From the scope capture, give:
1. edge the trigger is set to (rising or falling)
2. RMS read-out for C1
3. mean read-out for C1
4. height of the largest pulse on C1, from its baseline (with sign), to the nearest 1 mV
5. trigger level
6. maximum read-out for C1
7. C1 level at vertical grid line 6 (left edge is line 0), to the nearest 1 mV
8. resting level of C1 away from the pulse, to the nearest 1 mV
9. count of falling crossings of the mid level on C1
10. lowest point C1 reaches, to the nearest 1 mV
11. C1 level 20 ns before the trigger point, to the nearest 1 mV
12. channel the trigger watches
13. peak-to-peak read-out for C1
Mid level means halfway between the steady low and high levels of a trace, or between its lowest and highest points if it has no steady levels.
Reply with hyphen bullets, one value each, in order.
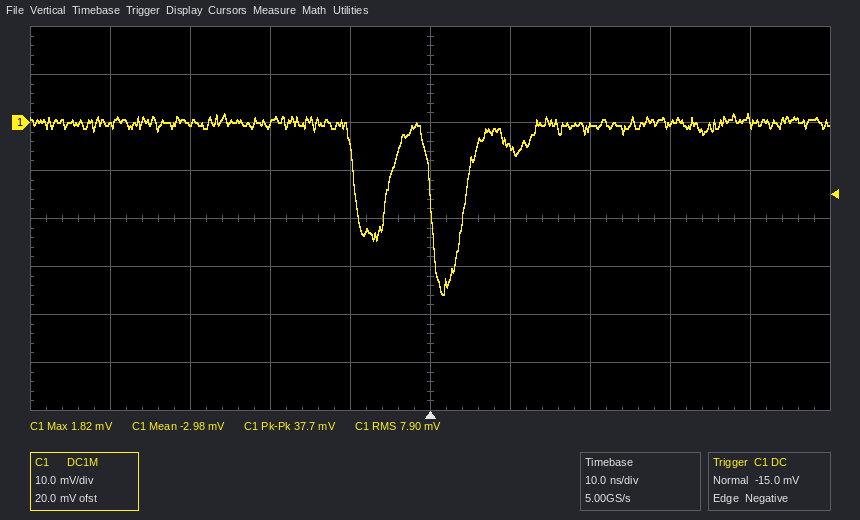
- falling
- 7.90 mV
- -2.98 mV
- -36 mV
- -15.0 mV
- 1.82 mV
- -5 mV
- 0 mV
- 2
- -36 mV
- 0 mV
- C1
- 37.7 mV
